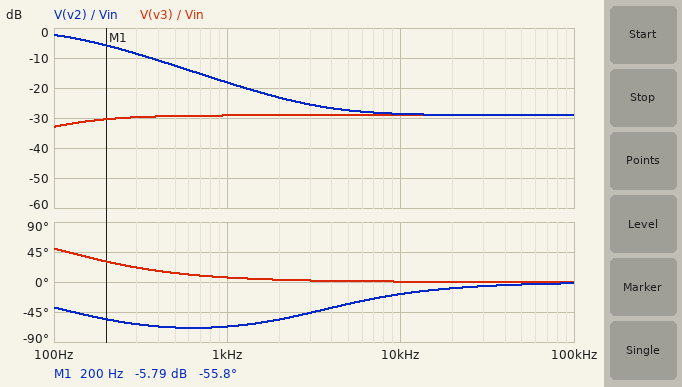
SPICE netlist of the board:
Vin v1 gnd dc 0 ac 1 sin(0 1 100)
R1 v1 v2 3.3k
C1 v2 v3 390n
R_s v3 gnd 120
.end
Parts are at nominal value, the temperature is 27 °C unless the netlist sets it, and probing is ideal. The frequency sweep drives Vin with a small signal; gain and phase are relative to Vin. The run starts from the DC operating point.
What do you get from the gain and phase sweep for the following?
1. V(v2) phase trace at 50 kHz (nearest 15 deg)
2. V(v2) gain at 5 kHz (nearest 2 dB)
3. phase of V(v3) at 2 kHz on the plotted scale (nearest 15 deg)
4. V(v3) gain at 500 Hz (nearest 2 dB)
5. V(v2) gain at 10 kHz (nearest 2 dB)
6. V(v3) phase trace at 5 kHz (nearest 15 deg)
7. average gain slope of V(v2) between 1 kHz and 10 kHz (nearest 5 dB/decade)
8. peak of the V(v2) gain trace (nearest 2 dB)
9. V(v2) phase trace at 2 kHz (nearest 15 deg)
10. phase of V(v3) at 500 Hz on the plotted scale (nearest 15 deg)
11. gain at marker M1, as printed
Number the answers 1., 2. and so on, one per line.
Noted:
1. 0 deg
2. -28 dB
3. 0 deg
4. -30 dB
5. -28 dB
6. 0 deg
7. -10 dB/decade
8. -2 dB
9. -60 deg
10. 15 deg
11. -5.79 dB
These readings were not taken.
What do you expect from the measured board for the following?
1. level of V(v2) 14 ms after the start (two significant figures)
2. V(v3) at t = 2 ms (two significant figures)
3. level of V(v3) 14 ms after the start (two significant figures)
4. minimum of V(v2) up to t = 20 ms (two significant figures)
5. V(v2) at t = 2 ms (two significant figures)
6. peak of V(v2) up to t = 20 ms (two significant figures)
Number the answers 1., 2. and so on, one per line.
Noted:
1. 740 mV
2. 15 mV
3. -5.5 mV
4. -770 mV
5. 530 mV
6. 800 mV
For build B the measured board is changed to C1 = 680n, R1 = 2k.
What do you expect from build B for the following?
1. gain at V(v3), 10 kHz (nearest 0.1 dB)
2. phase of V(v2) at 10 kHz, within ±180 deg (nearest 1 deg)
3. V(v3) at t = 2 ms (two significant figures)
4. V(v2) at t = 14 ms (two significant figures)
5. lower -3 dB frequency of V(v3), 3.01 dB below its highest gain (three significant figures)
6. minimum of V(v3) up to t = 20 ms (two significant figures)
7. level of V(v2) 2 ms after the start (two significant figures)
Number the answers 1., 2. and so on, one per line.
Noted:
1. -24.9 dB
2. -10 deg
3. 26 mV
4. 720 mV
5. 110 Hz
6. -38 mV
7. 520 mV
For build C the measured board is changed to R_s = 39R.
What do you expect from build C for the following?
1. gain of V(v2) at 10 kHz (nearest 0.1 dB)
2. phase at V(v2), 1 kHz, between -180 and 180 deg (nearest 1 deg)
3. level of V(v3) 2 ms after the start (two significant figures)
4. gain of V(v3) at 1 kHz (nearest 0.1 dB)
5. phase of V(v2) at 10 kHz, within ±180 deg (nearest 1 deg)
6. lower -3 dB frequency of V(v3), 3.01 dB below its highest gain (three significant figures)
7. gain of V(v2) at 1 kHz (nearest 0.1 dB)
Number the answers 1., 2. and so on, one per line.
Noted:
1. -35.4 dB
2. -78 deg
3. 5.0 mV
4. -38.7 dB
5. -46 deg
6. 122 Hz
7. -18.3 dB
